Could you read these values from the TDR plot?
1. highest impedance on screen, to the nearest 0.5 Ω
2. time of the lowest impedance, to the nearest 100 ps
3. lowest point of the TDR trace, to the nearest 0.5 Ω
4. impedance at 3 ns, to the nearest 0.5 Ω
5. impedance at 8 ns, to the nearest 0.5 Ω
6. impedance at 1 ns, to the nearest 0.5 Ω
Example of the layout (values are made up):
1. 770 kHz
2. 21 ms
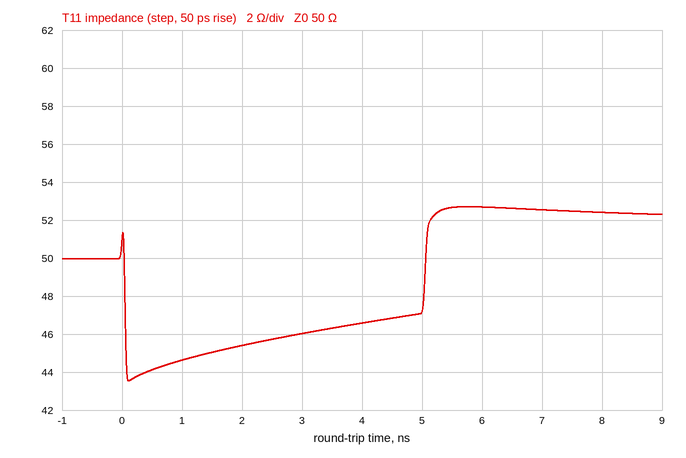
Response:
1. 52.5 Ω
2. 100 ps
3. 43.5 Ω
4. 46.0 Ω
5. 52.5 Ω
6. 44.5 Ω
